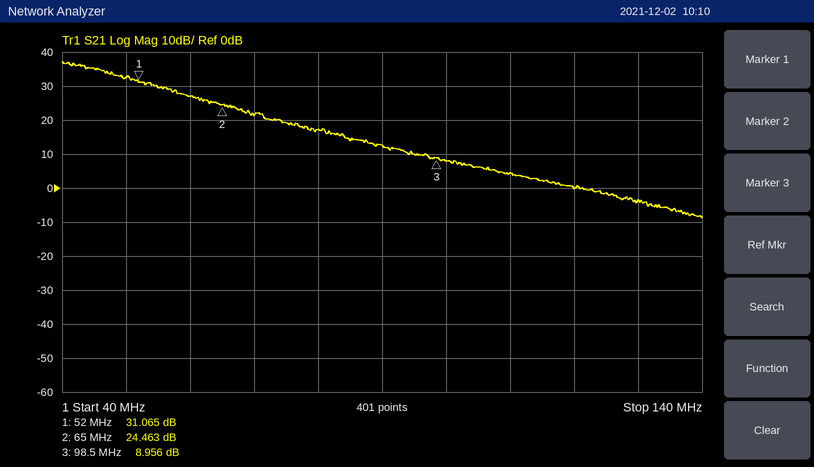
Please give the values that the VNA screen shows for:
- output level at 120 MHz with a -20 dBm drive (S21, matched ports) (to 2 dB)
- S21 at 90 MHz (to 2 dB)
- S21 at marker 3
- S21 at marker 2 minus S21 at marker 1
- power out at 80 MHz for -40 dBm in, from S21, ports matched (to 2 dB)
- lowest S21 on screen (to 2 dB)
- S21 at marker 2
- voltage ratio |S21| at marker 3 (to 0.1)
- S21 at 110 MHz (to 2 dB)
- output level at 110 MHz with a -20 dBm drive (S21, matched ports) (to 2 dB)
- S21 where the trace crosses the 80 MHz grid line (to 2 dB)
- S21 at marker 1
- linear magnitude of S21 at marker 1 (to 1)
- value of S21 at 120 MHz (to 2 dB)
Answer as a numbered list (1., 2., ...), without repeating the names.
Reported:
1. -20 dBm
2. 12 dB
3. 8.956 dB
4. -6.602 dB
5. -22 dBm
6. -8 dB
7. 24.463 dB
8. 2.8
9. 4 dB
10. -16 dBm
11. 18 dB
12. 31.065 dB
13. 36
14. 0 dB
